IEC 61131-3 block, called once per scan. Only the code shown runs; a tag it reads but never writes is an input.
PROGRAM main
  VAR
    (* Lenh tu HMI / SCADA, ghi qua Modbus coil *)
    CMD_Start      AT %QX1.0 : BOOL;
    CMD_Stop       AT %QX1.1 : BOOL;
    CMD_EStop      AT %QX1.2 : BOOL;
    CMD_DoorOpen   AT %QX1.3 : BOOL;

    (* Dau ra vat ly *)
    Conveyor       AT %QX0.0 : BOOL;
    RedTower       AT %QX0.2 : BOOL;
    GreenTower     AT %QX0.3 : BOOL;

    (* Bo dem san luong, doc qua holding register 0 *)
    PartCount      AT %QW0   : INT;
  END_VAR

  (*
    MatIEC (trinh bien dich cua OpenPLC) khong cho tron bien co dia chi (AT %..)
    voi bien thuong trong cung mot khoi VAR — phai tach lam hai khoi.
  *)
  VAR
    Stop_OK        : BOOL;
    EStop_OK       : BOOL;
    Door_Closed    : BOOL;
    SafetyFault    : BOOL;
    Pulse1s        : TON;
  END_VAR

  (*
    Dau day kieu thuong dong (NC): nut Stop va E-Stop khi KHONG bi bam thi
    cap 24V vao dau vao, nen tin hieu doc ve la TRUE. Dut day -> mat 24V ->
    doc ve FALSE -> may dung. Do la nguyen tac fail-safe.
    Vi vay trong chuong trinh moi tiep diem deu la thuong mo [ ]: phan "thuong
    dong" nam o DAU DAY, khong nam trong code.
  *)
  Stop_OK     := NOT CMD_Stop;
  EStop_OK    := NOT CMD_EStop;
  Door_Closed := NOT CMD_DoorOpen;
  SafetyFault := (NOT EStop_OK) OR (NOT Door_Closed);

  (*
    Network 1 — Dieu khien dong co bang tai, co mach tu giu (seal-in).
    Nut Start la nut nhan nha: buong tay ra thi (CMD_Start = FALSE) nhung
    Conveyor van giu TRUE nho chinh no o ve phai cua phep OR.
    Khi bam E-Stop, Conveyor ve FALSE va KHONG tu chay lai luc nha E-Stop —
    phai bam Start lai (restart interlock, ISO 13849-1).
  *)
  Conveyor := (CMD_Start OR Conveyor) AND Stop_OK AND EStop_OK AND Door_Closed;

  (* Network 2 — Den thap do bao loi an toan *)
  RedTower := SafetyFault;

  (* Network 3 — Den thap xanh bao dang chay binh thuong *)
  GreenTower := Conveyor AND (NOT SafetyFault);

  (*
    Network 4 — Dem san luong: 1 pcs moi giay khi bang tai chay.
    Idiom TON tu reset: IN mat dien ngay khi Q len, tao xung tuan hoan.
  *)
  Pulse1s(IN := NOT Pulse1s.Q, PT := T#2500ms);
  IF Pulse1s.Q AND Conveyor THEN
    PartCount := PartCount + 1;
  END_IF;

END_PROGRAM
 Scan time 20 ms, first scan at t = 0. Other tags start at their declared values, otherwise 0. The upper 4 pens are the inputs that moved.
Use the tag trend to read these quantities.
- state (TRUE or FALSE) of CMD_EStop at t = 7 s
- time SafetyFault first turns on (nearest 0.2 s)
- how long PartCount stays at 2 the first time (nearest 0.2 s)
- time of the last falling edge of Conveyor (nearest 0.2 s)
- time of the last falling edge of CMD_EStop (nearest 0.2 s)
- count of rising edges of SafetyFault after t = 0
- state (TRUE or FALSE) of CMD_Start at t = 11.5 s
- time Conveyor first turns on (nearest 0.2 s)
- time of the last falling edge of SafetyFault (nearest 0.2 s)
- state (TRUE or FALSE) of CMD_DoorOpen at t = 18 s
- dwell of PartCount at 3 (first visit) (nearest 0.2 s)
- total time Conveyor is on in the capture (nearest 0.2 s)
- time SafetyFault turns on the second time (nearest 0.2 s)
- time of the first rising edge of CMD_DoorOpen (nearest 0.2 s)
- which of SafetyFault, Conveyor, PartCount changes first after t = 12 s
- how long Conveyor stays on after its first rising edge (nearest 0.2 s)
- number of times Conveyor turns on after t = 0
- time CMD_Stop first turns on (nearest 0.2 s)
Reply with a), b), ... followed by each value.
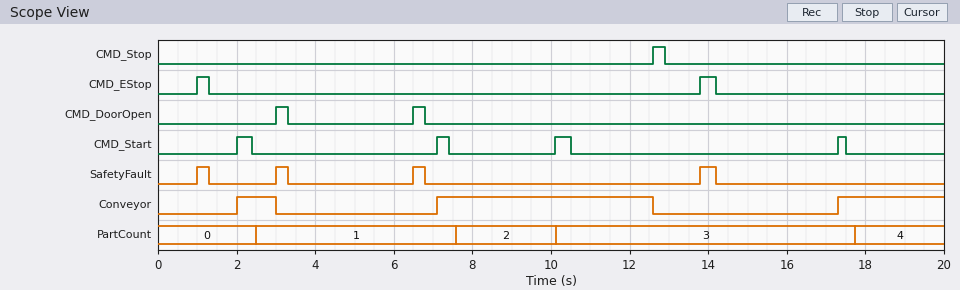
a) FALSE
b) 1.0 s
c) 2.6 s
d) 12.6 s
e) 14.2 s
f) 4
g) FALSE
h) 2.0 s
i) 14.2 s
j) FALSE
k) 7.6 s
l) 9.2 s
m) 3.0 s
n) 3.0 s
o) Conveyor
p) 1.0 s
q) 3
r) 12.6 s
